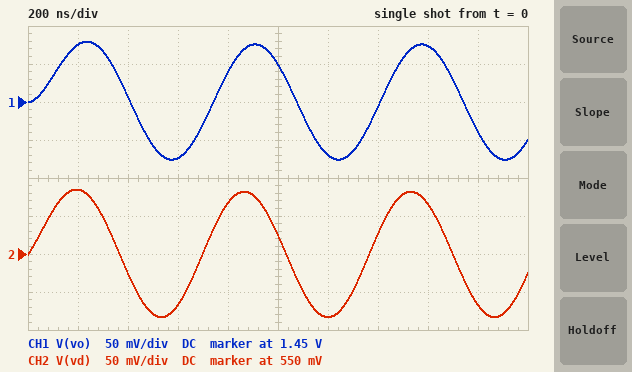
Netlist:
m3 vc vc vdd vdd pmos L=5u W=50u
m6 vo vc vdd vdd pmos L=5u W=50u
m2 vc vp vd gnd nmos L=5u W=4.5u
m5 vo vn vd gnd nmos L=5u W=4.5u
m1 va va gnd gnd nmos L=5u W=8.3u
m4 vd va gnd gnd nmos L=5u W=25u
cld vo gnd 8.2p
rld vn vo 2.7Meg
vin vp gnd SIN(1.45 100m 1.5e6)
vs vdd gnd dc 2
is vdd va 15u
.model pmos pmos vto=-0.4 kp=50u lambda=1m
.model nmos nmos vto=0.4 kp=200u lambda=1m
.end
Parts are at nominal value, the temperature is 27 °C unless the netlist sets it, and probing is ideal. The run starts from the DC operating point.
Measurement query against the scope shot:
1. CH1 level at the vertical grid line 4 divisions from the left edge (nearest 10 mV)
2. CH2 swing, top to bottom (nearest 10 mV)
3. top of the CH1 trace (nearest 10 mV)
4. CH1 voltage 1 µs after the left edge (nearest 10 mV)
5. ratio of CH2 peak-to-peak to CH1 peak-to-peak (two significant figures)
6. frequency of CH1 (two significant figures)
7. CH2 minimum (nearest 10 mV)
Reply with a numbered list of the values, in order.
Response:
1. 1.49 V
2. 170 mV
3. 1.53 V
4. 1.50 V
5. 1.1
6. 1.5 MHz
7. 470 mV
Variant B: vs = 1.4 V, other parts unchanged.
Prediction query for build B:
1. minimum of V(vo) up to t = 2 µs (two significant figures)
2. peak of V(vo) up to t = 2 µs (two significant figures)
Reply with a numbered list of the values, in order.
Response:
1. 1.2 V
2. 1.3 V
